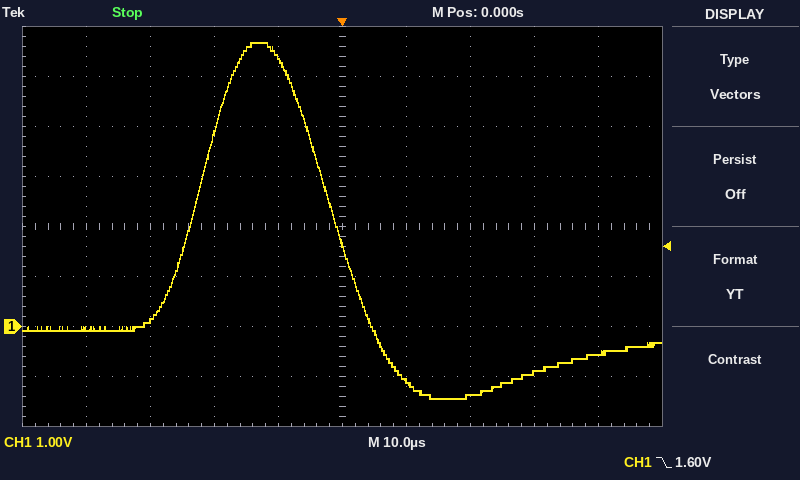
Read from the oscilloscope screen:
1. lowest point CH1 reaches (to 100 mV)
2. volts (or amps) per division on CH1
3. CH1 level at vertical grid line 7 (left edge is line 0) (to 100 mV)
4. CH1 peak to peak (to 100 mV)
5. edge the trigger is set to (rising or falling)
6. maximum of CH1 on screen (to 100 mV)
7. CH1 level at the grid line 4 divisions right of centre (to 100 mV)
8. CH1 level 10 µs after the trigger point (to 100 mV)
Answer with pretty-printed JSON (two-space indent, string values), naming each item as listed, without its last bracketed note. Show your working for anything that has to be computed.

{
  "lowest point CH1 reaches": "-1.4 V",
  "volts (or amps) per division on CH1": "1 V",
  "CH1 level at vertical grid line 7 (left edge is line 0)": "-1.4 V",
  "CH1 peak to peak": "5.7 V − (-1.4 V) = 7.1 V",
  "edge the trigger is set to": "falling",
  "maximum of CH1 on screen": "5.7 V",
  "CH1 level at the grid line 4 divisions right of centre": "-600 mV",
  "CH1 level 10 µs after the trigger point": "-1.1 V"
}
